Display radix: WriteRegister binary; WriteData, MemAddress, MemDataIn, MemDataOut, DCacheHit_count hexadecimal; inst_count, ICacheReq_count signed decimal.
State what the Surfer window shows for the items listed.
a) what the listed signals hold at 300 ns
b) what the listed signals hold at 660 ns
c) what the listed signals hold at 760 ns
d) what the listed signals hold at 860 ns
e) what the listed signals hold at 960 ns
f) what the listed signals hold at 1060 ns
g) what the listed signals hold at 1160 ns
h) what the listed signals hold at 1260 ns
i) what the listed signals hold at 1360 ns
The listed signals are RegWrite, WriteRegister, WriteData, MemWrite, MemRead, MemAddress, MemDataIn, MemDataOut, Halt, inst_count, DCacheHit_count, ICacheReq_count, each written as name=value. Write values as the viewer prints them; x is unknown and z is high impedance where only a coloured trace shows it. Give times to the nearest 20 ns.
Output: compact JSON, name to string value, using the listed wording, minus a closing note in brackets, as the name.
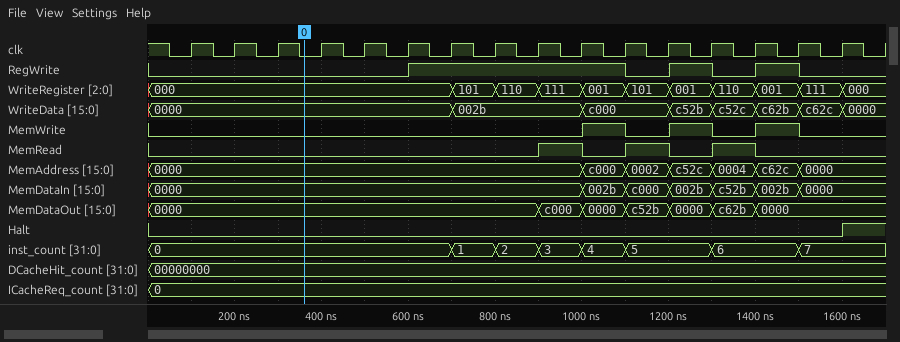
{"what the listed signals hold at 300 ns": "RegWrite=0, WriteRegister=000, WriteData=0000, MemWrite=0, MemRead=0, MemAddress=0000, MemDataIn=0000, MemDataOut=0000, Halt=0, inst_count=0, DCacheHit_count=00000000, ICacheReq_count=0", "what the listed signals hold at 660 ns": "RegWrite=1, WriteRegister=000, WriteData=0000, MemWrite=0, MemRead=0, MemAddress=0000, MemDataIn=0000, MemDataOut=0000, Halt=0, inst_count=0, DCacheHit_count=00000000, ICacheReq_count=0", "what the listed signals hold at 760 ns": "RegWrite=1, WriteRegister=101, WriteData=002b, MemWrite=0, MemRead=0, MemAddress=0000, MemDataIn=0000, MemDataOut=0000, Halt=0, inst_count=1, DCacheHit_count=00000000, ICacheReq_count=0", "what the listed signals hold at 860 ns": "RegWrite=1, WriteRegister=110, WriteData=002b, MemWrite=0, MemRead=0, MemAddress=0000, MemDataIn=0000, MemDataOut=0000, Halt=0, inst_count=2, DCacheHit_count=00000000, ICacheReq_count=0", "what the listed signals hold at 960 ns": "RegWrite=1, WriteRegister=111, WriteData=002b, MemWrite=0, MemRead=1, MemAddress=0000, MemDataIn=0000, MemDataOut=c000, Halt=0, inst_count=3, DCacheHit_count=00000000, ICacheReq_count=0", "what the listed signals hold at 1060 ns": "RegWrite=1, WriteRegister=001, WriteData=c000, MemWrite=1, MemRead=0, MemAddress=c000, MemDataIn=002b, MemDataOut=0000, Halt=0, inst_count=4, DCacheHit_count=00000000, ICacheReq_count=0", "what the listed signals hold at 1160 ns": "RegWrite=0, WriteRegister=101, WriteData=c000, MemWrite=0, MemRead=1, MemAddress=0002, MemDataIn=c000, MemDataOut=c52b, Halt=0, inst_count=5, DCacheHit_count=00000000, ICacheReq_count=0", "what the listed signals hold at 1260 ns": "RegWrite=1, WriteRegister=001, WriteData=c52b, MemWrite=1, MemRead=0, MemAddress=c52c, MemDataIn=002b, MemDataOut=0000, Halt=0, inst_count=5, DCacheHit_count=00000000, ICacheReq_count=0", "what the listed signals hold at 1360 ns": "RegWrite=0, WriteRegister=110, WriteData=c52c, MemWrite=0, MemRead=1, MemAddress=0004, MemDataIn=c52b, MemDataOut=c62b, Halt=0, inst_count=6, DCacheHit_count=00000000, ICacheReq_count=0"}
